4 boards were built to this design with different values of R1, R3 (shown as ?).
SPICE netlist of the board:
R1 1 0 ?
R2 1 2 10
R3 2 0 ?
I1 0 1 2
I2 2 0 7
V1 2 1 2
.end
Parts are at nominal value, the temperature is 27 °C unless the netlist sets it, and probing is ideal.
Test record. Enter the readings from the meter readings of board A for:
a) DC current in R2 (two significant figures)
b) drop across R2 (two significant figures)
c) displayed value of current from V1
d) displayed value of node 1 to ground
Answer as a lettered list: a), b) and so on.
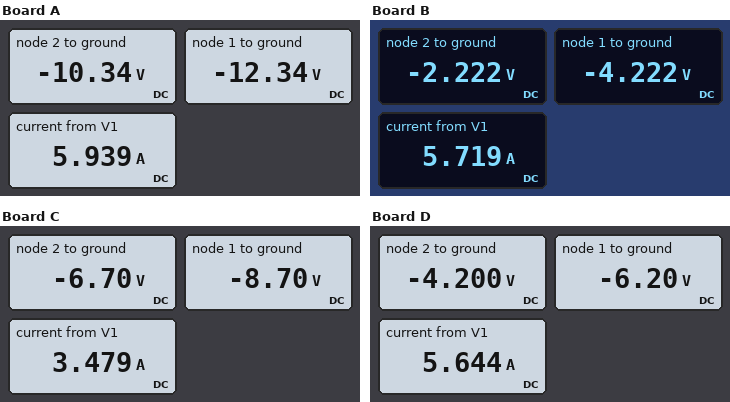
a) 200 mA
b) 2.0 V
c) 5.939 A
d) -12.34 V
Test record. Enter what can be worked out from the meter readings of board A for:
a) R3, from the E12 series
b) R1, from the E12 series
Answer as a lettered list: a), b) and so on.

a) 8.2 Ω
b) 3.3 Ω
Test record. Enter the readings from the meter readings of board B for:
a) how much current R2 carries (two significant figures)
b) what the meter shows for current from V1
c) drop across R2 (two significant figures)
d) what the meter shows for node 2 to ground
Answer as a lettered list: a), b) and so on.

a) 200 mA
b) 5.719 A
c) 2.0 V
d) -2.222 V
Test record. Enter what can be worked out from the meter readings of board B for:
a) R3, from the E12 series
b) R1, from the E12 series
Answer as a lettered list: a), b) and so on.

a) 1.5 Ω
b) 1.2 Ω
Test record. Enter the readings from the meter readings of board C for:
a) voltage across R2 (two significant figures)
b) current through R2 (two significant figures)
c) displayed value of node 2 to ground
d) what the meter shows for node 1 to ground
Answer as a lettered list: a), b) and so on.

a) 2.0 V
b) 200 mA
c) -6.70 V
d) -8.70 V
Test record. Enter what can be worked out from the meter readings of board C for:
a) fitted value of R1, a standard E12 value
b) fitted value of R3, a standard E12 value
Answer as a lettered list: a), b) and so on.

a) 6.8 Ω
b) 1.8 Ω
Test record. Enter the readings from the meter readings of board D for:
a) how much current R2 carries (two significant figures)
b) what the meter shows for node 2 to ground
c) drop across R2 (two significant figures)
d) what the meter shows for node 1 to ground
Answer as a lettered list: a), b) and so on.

a) 200 mA
b) -4.200 V
c) 2.0 V
d) -6.20 V
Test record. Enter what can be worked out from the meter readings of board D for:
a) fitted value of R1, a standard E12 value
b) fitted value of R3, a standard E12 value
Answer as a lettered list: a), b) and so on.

a) 1.8 Ω
b) 2.7 Ω
